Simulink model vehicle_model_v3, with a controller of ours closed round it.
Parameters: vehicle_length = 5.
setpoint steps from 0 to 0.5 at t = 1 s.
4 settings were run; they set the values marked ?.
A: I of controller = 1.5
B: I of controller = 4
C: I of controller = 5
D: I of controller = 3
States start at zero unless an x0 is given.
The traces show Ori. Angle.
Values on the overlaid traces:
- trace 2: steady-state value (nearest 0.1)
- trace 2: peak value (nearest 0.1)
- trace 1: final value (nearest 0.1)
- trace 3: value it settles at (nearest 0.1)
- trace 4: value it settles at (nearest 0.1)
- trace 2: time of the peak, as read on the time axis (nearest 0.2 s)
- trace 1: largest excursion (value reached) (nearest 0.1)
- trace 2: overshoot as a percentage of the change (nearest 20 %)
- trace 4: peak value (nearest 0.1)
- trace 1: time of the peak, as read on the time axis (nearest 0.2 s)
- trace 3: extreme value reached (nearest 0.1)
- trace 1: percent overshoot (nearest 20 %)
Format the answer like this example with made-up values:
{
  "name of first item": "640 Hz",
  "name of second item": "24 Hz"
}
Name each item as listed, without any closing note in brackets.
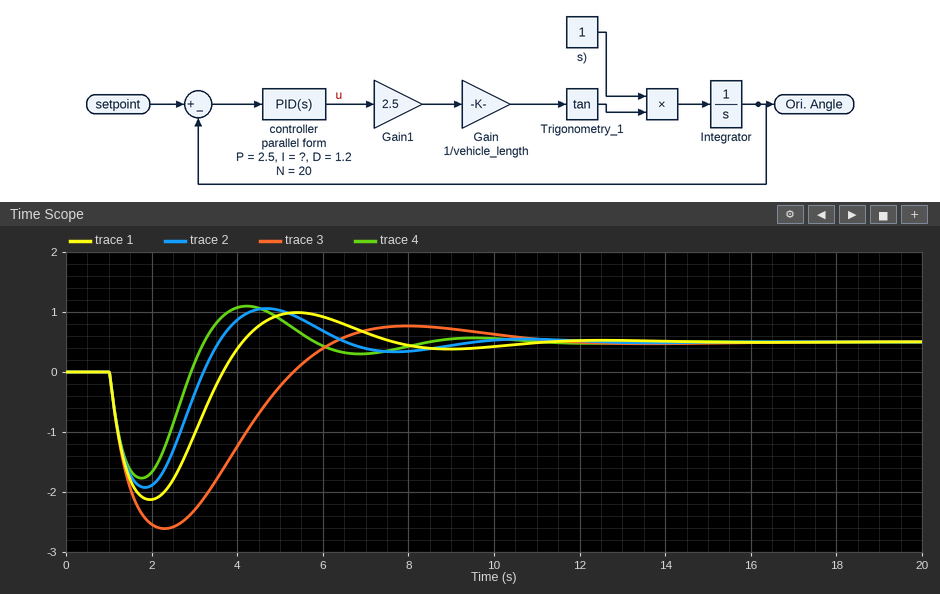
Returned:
{
  "trace 2: steady-state value": "0.5",
  "trace 2: peak value": "1.1",
  "trace 1: final value": "0.5",
  "trace 3: value it settles at": "0.5",
  "trace 4: value it settles at": "0.5",
  "trace 2: time of the peak, as read on the time axis": "4.6 s",
  "trace 1: largest excursion (value reached)": "1.0",
  "trace 2: overshoot as a percentage of the change": "120 %",
  "trace 4: peak value": "1.1",
  "trace 1: time of the peak, as read on the time axis": "5.4 s",
  "trace 3: extreme value reached": "-2.6",
  "trace 1: percent overshoot": "100 %"
}
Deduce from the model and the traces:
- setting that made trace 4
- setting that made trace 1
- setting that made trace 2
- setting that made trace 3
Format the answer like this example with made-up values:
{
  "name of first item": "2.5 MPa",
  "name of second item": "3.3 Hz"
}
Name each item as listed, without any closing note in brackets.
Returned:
{
  "setting that made trace 4": "C",
  "setting that made trace 1": "D",
  "setting that made trace 2": "B",
  "setting that made trace 3": "A"
}
